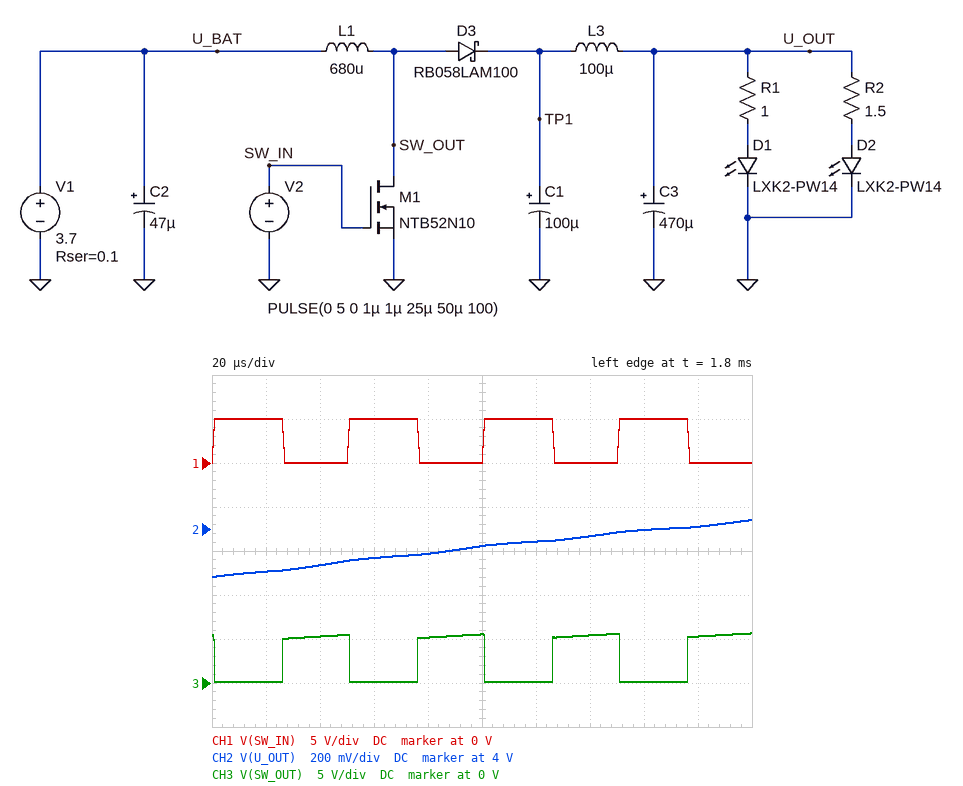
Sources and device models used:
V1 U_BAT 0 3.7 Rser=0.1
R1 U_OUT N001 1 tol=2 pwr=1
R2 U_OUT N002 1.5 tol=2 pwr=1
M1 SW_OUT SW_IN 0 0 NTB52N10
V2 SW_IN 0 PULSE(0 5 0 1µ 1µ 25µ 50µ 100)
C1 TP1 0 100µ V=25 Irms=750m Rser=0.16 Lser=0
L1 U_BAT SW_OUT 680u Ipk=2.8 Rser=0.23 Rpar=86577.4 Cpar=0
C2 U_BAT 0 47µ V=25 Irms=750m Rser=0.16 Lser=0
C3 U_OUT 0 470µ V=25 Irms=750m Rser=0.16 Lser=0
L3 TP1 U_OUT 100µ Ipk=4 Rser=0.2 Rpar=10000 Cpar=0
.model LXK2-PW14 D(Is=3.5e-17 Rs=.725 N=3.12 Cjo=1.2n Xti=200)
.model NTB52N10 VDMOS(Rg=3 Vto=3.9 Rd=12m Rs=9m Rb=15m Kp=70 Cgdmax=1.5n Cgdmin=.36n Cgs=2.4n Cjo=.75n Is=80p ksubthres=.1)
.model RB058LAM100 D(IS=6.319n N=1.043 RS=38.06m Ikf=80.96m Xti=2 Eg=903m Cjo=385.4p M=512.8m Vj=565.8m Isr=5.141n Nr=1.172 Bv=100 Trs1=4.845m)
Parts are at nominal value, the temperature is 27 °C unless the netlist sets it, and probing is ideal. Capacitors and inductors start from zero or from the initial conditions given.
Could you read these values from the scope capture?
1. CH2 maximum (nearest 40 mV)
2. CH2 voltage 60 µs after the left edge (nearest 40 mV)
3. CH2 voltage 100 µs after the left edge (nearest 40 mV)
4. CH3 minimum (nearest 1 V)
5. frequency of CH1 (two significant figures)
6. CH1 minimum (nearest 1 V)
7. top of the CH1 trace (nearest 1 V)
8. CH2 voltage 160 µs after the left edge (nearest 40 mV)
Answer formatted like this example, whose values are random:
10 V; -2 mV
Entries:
4.04 V; 3.88 V; 3.92 V; 0 V; 20 kHz; 0 V; 5 V; 4.00 V
